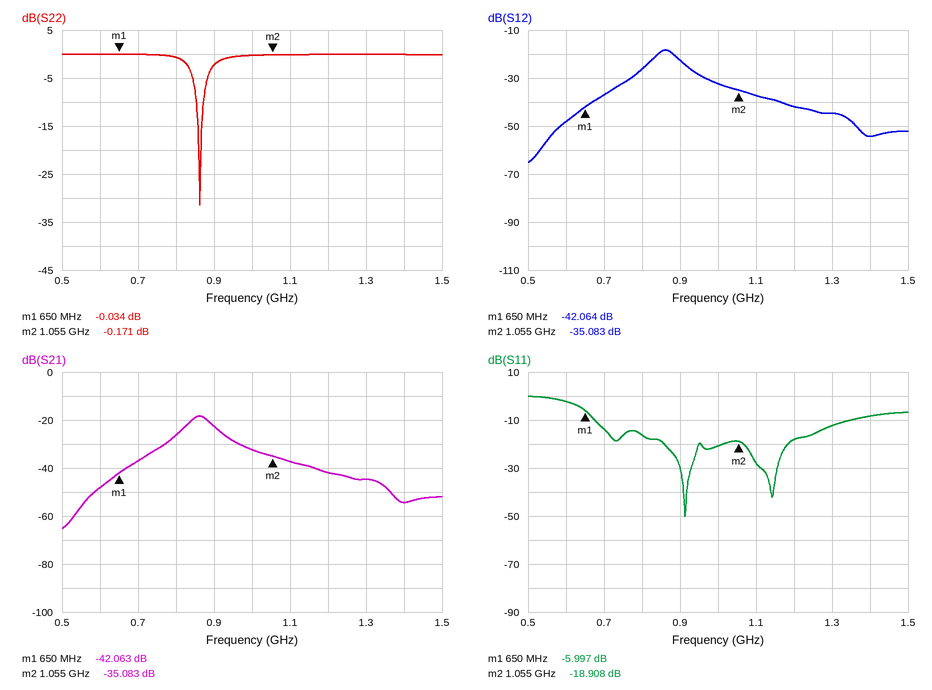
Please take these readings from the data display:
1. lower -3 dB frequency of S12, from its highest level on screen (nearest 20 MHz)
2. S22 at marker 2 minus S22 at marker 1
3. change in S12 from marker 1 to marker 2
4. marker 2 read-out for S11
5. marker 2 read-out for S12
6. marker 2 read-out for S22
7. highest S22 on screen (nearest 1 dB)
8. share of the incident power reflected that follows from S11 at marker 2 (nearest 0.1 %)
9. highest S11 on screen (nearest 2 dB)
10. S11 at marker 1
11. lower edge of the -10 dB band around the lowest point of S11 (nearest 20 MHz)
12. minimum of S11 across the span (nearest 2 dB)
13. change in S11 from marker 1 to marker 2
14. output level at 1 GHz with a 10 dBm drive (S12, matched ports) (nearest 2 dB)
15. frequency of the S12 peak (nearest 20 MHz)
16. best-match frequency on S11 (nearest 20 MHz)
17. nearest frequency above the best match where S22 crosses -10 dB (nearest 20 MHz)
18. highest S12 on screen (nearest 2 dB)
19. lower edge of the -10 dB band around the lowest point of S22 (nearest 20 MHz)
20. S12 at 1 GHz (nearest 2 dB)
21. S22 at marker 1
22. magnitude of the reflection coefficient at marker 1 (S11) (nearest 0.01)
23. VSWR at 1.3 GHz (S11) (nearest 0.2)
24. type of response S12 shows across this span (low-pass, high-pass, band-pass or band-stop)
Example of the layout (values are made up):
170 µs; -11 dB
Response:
840 MHz; -0.137 dB; 6.981 dB; -18.908 dB; -35.083 dB; -0.171 dB; 0 dB; 1.3 %; 0 dB; -5.997 dB; 680 MHz; -50 dB; -12.911 dB; -22 dBm; 860 MHz; 920 MHz; 880 MHz; -18 dB; 860 MHz; -32 dB; -0.034 dB; 0.50; 1.6; band-pass
